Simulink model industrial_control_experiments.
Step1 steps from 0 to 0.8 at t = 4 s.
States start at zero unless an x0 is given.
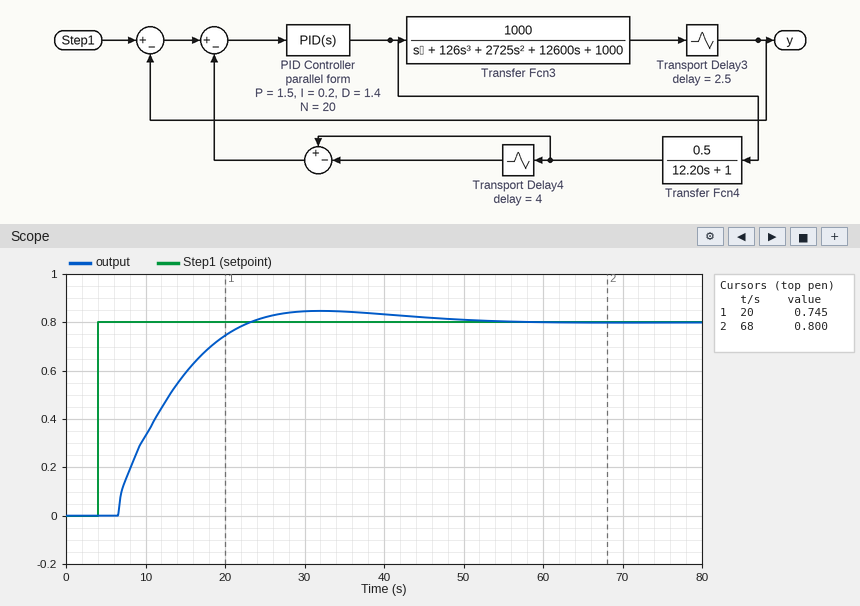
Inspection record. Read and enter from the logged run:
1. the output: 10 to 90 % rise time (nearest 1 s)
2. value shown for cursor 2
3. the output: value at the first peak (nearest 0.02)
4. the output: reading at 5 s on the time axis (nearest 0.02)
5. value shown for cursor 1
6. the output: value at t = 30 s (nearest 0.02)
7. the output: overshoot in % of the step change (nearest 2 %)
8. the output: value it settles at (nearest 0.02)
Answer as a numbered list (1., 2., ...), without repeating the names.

1. 12 s
2. 0.800
3. 0.84
4. 0.00
5. 0.745
6. 0.84
7. 6 %
8. 0.80
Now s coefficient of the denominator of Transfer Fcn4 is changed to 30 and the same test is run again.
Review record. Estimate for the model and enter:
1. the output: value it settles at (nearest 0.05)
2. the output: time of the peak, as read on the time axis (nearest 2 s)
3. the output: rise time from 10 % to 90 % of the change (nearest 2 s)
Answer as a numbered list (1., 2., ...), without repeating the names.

1. 0.80
2. 28 s
3. 10 s
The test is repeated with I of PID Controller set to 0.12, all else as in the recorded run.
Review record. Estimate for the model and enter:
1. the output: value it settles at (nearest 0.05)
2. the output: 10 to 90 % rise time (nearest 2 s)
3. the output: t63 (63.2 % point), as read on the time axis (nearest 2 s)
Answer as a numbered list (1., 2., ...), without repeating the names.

1. 0.80
2. 18 s
3. 14 s
